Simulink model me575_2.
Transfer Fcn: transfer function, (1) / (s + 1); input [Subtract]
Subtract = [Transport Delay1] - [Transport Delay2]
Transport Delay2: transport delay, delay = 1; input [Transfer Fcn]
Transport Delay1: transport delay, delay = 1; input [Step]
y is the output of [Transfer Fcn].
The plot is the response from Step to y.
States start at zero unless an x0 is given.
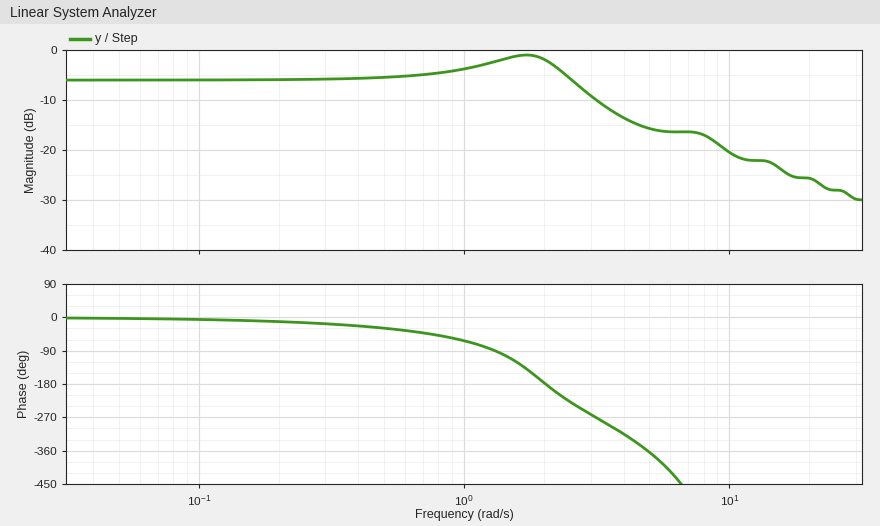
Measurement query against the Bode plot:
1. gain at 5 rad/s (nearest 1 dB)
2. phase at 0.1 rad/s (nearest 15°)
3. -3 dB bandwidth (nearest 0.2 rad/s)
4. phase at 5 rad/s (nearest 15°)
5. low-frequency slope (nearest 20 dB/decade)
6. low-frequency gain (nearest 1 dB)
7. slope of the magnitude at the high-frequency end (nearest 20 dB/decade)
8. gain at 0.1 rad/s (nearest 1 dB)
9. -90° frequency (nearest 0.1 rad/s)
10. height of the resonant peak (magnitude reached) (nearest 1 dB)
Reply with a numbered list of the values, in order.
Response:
1. -16 dB
2. 0°
3. 3.0 rad/s
4. -360°
5. 0 dB/decade
6. -6 dB
7. -20 dB/decade
8. -6 dB
9. 1.3 rad/s
10. -1 dB
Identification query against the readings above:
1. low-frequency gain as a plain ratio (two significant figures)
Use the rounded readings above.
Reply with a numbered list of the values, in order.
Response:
1. 0.50
